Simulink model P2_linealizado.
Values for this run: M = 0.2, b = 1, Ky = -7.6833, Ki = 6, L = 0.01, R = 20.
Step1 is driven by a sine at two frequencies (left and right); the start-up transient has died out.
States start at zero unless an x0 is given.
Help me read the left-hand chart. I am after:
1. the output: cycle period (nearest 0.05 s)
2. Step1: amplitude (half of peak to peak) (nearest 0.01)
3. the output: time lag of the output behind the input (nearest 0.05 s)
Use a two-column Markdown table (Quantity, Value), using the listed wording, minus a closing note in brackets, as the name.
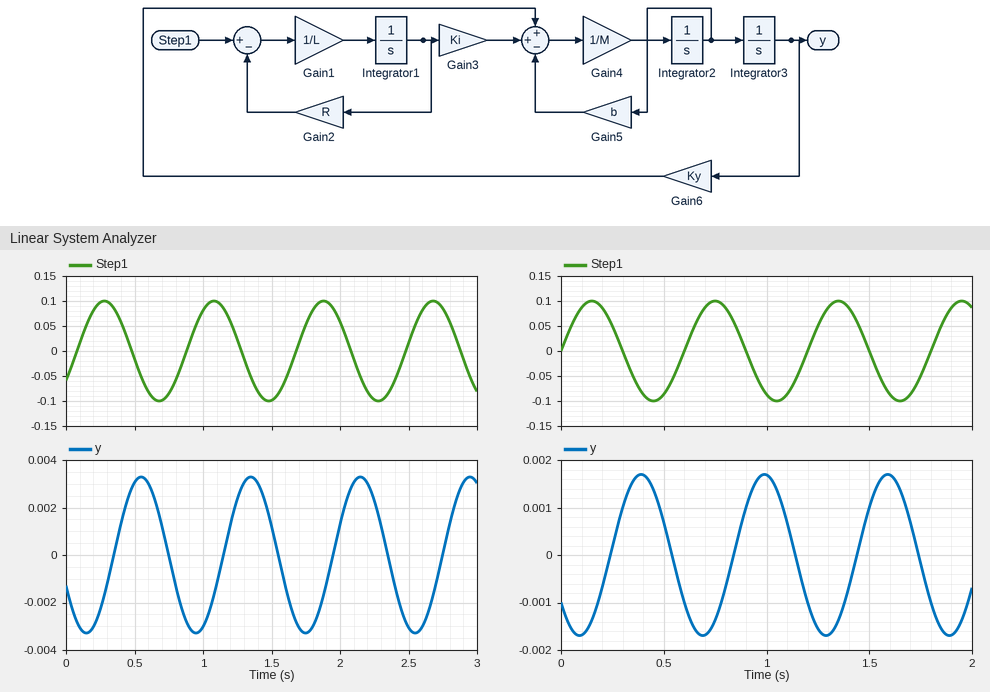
| Quantity | Value |
|---|---|
| the output: cycle period | 0.80 s |
| Step1: amplitude (half of peak to peak) | 0.10 |
| the output: time lag of the output behind the input | 0.25 s |
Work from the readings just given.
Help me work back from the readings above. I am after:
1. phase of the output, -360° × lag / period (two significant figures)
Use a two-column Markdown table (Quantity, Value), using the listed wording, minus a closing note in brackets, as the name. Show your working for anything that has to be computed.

| Quantity | Value |
|---|---|
| phase of the output, -360° × lag / period | -360 × 0.25 / 0.8 = -110° |
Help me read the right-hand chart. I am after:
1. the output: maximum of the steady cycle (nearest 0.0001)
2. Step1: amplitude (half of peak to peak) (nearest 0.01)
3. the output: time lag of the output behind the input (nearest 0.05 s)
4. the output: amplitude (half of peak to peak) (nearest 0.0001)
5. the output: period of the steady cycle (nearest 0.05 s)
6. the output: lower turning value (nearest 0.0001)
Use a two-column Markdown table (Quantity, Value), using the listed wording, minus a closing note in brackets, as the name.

| Quantity | Value |
|---|---|
| the output: maximum of the steady cycle | 0.0017 |
| Step1: amplitude (half of peak to peak) | 0.10 |
| the output: time lag of the output behind the input | 0.25 s |
| the output: amplitude (half of peak to peak) | 0.0017 |
| the output: period of the steady cycle | 0.60 s |
| the output: lower turning value | -0.0017 |
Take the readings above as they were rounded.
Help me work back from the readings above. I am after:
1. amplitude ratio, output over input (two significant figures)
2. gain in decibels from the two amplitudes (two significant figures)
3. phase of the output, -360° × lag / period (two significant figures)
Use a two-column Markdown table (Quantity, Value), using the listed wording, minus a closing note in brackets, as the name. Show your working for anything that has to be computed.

| Quantity | Value |
|---|---|
| amplitude ratio, output over input | 0.0017 / 0.1 = 0.017 |
| gain in decibels from the two amplitudes | 20 log10(0.0017 / 0.1) = -35 dB |
| phase of the output, -360° × lag / period | -360 × 0.25 / 0.6 = -150° |
